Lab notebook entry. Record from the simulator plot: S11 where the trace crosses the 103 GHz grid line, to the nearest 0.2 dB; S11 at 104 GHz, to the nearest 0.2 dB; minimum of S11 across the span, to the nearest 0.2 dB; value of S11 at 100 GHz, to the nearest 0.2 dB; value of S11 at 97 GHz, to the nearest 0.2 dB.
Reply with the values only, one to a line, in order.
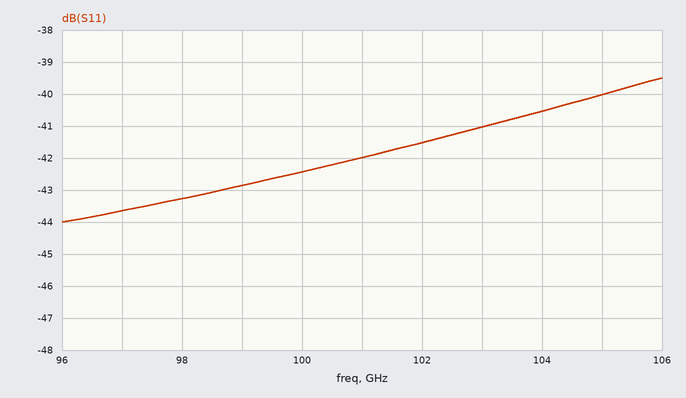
-41.0 dB
-40.6 dB
-44.0 dB
-42.4 dB
-43.6 dB
